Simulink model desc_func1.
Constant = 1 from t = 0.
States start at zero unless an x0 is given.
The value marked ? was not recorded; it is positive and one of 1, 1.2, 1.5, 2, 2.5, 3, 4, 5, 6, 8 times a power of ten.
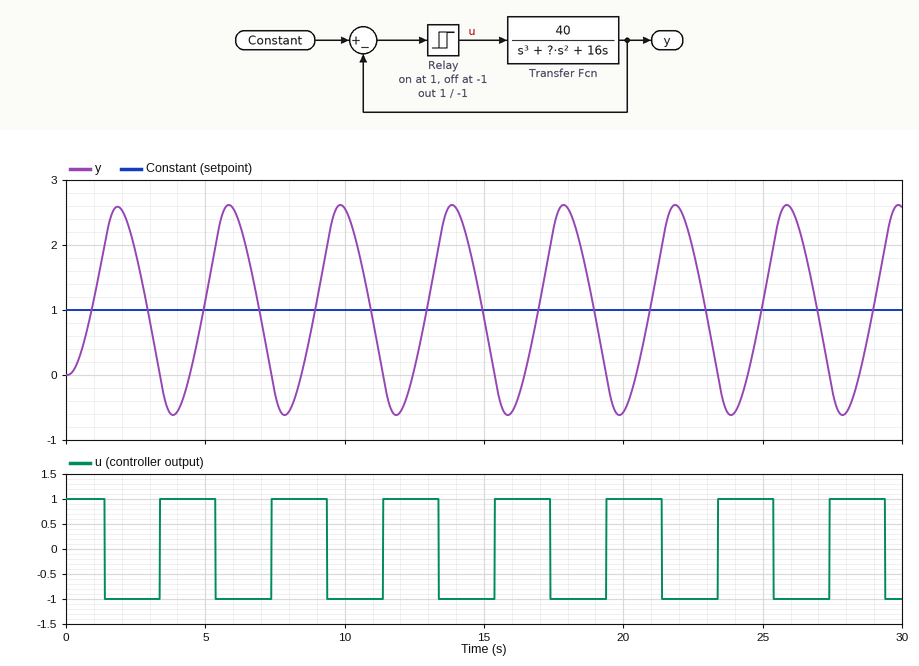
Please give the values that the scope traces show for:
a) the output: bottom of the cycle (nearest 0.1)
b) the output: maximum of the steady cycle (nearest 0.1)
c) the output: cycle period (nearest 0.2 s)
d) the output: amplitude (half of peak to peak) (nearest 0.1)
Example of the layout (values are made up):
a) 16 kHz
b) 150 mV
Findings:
a) -0.6
b) 2.6
c) 4.0 s
d) 1.6
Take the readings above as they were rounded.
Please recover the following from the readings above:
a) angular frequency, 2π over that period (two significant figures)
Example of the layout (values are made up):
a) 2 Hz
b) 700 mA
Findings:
a) 1.6 rad/s
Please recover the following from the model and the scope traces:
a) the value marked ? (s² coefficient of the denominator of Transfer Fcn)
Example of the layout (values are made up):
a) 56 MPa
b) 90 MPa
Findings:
a) 10
